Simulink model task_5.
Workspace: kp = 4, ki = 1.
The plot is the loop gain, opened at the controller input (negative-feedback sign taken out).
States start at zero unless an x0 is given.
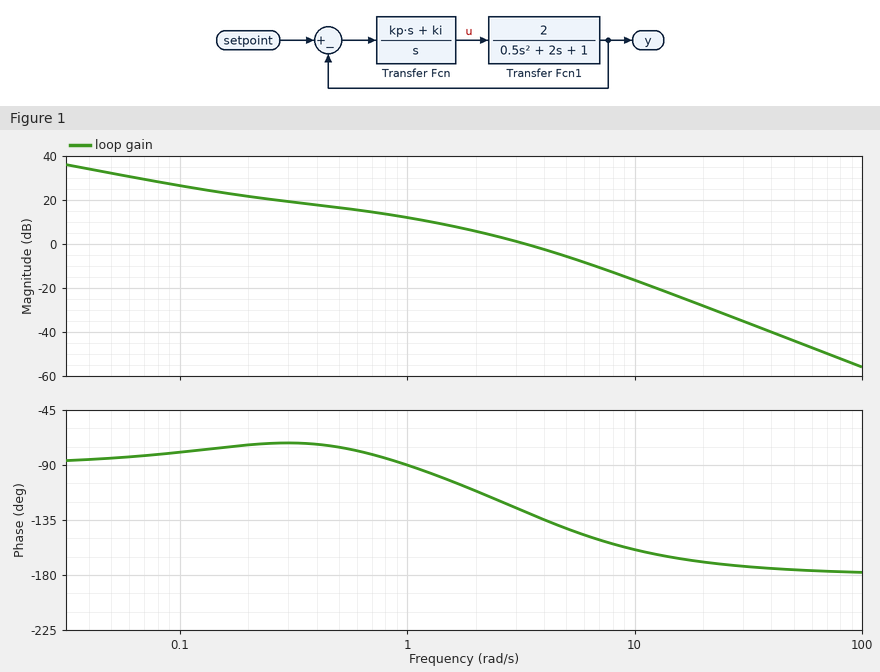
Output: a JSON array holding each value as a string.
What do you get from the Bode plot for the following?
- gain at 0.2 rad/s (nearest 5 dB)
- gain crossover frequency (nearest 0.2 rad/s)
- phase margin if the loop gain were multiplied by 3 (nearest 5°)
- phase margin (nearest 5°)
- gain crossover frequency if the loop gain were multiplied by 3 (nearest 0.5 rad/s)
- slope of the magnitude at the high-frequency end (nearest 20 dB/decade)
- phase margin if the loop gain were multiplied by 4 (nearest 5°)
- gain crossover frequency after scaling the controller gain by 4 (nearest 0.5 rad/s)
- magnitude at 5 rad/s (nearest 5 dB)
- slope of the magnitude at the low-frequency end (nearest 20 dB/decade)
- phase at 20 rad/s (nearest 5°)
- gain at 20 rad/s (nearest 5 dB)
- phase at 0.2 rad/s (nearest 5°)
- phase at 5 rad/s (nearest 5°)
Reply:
["20 dB", "3.4 rad/s", "30°", "50°", "6.5 rad/s", "-40 dB/decade", "25°", "7.5 rad/s", "-5 dB", "-20 dB/decade", "-170°", "-30 dB", "-75°", "-140°"]
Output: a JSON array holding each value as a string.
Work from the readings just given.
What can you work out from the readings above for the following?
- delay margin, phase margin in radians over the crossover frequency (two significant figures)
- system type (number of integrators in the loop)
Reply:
["0.26 s", "1"]
